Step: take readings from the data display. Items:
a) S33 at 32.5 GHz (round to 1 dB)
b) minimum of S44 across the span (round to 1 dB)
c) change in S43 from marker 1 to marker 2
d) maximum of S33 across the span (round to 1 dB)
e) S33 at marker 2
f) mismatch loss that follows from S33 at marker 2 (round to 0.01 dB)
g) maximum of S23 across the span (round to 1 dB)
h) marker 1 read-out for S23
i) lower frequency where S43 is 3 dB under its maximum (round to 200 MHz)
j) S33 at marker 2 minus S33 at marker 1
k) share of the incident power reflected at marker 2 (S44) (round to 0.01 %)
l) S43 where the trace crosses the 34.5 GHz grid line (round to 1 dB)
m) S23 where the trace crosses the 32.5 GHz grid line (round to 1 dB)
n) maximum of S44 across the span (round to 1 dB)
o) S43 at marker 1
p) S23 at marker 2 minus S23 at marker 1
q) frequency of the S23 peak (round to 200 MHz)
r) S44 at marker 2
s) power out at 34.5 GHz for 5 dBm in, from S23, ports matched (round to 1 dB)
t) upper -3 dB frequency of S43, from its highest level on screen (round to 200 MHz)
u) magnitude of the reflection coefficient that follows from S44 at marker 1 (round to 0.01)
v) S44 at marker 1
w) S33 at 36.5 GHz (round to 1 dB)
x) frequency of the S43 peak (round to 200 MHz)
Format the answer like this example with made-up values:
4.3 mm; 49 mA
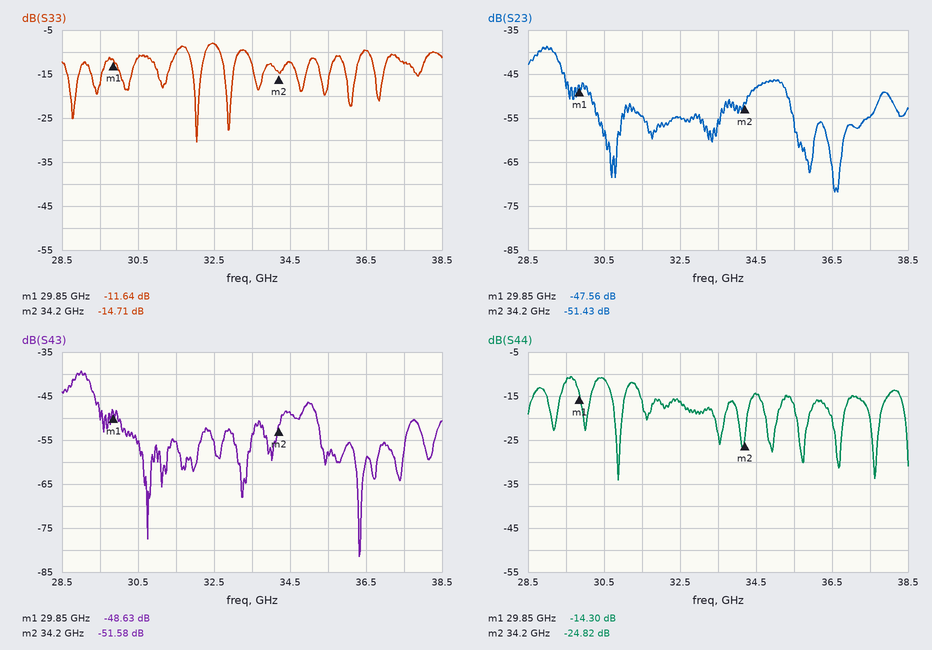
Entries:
-8 dB; -34 dB; -2.95 dB; -8 dB; -14.71 dB; 0.15 dB; -39 dB; -47.56 dB; 28.8 GHz; -3.07 dB; 0.33 %; -49 dB; -55 dB; -11 dB; -48.63 dB; -3.87 dB; 29.0 GHz; -24.82 dB; -43 dBm; 29.2 GHz; 0.19; -14.30 dB; -10 dB; 29.0 GHz
